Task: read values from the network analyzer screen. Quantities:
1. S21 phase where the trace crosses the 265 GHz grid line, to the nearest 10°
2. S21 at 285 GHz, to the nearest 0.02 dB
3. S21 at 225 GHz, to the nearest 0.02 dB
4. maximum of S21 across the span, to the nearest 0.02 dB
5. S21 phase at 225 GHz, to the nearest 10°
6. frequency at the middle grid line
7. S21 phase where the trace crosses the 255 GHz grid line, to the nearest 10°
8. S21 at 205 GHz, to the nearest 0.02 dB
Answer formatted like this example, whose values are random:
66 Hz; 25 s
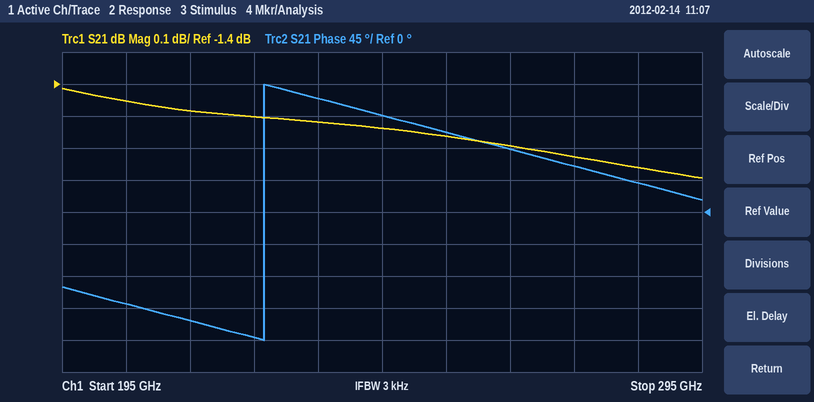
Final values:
90°; -1.66 dB; -1.50 dB; -1.42 dB; -180°; 245 GHz; 110°; -1.46 dB
